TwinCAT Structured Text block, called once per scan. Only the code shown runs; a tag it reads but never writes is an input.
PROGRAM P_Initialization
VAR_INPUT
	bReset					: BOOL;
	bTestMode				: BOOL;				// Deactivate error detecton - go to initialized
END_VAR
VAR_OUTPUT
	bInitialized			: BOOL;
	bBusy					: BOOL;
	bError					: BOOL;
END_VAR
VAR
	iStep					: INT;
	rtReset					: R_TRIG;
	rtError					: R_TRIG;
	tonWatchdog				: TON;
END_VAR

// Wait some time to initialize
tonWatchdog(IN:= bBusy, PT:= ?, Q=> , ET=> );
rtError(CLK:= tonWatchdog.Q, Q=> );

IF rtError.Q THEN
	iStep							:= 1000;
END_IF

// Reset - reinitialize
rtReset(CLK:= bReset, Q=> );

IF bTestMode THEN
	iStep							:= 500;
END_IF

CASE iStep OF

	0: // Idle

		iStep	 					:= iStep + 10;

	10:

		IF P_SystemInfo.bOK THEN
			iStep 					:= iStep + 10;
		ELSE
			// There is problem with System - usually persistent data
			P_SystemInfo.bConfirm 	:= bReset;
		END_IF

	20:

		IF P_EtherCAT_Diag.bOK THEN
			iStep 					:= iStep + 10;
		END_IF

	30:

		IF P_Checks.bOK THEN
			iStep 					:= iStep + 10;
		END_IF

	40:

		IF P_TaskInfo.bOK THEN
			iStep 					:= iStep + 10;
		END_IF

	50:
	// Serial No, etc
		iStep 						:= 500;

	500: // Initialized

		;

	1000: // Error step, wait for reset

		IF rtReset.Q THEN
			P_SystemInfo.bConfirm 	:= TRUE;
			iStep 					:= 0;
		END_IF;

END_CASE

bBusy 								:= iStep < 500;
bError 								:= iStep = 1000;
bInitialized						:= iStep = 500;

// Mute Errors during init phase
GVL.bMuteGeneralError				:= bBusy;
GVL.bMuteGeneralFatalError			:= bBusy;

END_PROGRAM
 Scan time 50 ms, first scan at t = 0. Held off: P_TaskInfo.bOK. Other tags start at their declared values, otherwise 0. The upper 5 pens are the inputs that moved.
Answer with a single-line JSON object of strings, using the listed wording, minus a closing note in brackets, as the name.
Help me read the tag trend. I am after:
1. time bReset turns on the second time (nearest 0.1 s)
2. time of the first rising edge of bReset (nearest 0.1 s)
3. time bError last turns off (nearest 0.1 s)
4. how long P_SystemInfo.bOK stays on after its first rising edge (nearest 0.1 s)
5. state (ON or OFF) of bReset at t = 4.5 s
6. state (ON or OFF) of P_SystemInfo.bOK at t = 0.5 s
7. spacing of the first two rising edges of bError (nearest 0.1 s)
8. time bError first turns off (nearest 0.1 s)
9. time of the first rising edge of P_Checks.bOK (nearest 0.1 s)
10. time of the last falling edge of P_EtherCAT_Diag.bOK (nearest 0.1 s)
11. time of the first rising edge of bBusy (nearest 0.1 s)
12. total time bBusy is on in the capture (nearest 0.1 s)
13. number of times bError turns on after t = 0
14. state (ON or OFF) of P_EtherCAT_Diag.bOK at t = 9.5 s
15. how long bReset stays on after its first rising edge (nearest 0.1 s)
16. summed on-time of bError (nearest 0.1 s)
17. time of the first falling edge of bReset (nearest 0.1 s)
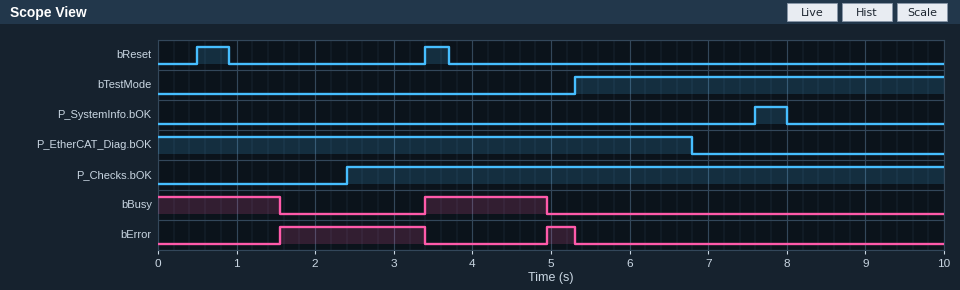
{"time bReset turns on the second time": "3.4 s", "time of the first rising edge of bReset": "0.5 s", "time bError last turns off": "5.3 s", "how long P_SystemInfo.bOK stays on after its first rising edge": "0.4 s", "state (ON or OFF) of bReset at t = 4.5 s": "OFF", "state (ON or OFF) of P_SystemInfo.bOK at t = 0.5 s": "OFF", "spacing of the first two rising edges of bError": "3.4 s", "time bError first turns off": "3.4 s", "time of the first rising edge of P_Checks.bOK": "2.4 s", "time of the last falling edge of P_EtherCAT_Diag.bOK": "6.8 s", "time of the first rising edge of bBusy": "3.4 s", "total time bBusy is on in the capture": "3.1 s", "number of times bError turns on after t = 0": "2", "state (ON or OFF) of P_EtherCAT_Diag.bOK at t = 9.5 s": "OFF", "how long bReset stays on after its first rising edge": "0.4 s", "summed on-time of bError": "2.2 s", "time of the first falling edge of bReset": "0.9 s"}
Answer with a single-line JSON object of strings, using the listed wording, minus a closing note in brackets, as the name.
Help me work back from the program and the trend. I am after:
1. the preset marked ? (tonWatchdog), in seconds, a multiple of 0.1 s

{"the preset marked ? (tonWatchdog), in seconds, a multiple of 0.1 s": "1.5 s"}
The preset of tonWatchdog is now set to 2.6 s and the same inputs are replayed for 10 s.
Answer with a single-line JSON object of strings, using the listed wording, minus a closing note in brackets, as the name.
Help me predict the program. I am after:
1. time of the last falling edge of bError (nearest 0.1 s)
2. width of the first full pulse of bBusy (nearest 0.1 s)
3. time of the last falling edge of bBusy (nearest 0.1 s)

{"time of the last falling edge of bError": "3.4 s", "width of the first full pulse of bBusy": "1.9 s", "time of the last falling edge of bBusy": "5.3 s"}
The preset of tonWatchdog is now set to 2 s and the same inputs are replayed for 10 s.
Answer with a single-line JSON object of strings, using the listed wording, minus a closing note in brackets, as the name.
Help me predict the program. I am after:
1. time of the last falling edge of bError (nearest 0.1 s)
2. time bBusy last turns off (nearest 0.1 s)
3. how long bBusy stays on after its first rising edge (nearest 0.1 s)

{"time of the last falling edge of bError": "3.4 s", "time bBusy last turns off": "5.3 s", "how long bBusy stays on after its first rising edge": "1.9 s"}
